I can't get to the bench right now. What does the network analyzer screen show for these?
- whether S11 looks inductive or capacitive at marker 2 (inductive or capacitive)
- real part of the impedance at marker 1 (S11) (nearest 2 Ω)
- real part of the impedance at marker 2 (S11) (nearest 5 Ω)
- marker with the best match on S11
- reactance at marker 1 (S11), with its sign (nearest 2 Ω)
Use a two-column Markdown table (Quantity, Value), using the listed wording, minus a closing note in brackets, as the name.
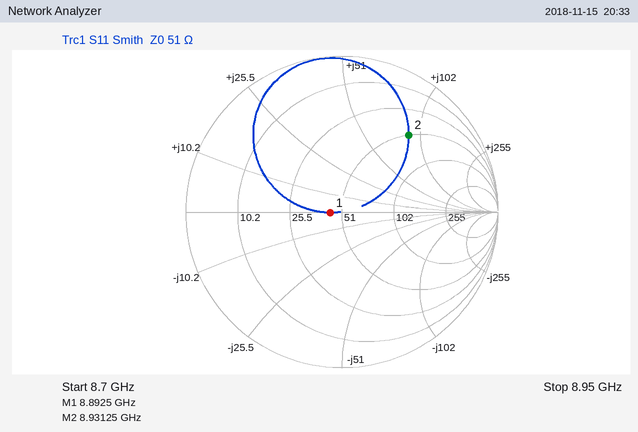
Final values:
| Quantity | Value |
|---|---|
| whether S11 looks inductive or capacitive at marker 2 | inductive |
| real part of the impedance at marker 1 (S11) | 44 Ω |
| real part of the impedance at marker 2 (S11) | 50 Ω |
| marker with the best match on S11 | marker 1 |
| reactance at marker 1 (S11), with its sign | 0 Ω |
